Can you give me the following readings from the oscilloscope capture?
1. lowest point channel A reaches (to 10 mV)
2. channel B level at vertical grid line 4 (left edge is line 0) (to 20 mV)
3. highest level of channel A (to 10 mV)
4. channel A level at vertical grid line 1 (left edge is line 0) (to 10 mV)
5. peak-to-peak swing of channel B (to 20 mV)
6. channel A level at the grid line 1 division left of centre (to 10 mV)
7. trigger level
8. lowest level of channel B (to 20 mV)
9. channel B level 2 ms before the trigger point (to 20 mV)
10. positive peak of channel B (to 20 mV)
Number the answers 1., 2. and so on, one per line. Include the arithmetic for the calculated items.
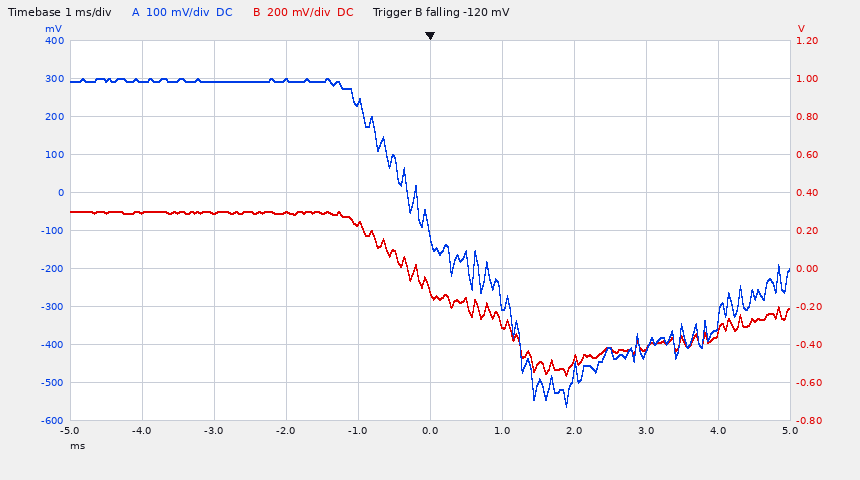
1. -560 mV
2. 240 mV
3. 300 mV
4. 290 mV
5. 300 mV − (-560 mV) = 860 mV
6. 240 mV
7. -120 mV
8. -560 mV
9. 300 mV
10. 300 mV
